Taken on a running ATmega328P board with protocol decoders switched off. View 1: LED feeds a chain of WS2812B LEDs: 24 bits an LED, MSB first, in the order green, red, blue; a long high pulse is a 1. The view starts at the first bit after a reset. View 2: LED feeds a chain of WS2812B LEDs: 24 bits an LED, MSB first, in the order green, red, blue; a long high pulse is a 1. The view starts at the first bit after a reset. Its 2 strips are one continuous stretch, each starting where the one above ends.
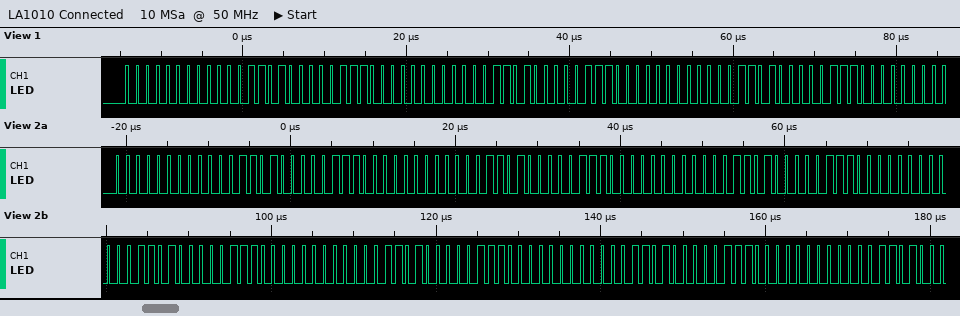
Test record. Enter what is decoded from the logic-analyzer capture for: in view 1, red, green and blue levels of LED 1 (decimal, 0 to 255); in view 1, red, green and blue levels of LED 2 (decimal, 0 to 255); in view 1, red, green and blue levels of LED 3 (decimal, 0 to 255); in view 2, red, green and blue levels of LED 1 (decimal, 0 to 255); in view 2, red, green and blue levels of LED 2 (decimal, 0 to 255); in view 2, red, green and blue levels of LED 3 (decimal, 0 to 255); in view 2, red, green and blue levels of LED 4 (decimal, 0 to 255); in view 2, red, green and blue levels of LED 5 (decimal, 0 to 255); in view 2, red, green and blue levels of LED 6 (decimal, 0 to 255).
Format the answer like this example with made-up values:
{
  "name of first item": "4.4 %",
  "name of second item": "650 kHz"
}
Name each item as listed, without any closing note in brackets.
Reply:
{
  "in view 1, red, green and blue levels of LED 1": "13, 0, 7",
  "in view 1, red, green and blue levels of LED 2": "13, 0, 7",
  "in view 1, red, green and blue levels of LED 3": "13, 0, 7",
  "in view 2, red, green and blue levels of LED 1": "13, 0, 7",
  "in view 2, red, green and blue levels of LED 2": "13, 0, 7",
  "in view 2, red, green and blue levels of LED 3": "13, 0, 7",
  "in view 2, red, green and blue levels of LED 4": "13, 0, 7",
  "in view 2, red, green and blue levels of LED 5": "13, 0, 7",
  "in view 2, red, green and blue levels of LED 6": "13, 0, 7"
}
